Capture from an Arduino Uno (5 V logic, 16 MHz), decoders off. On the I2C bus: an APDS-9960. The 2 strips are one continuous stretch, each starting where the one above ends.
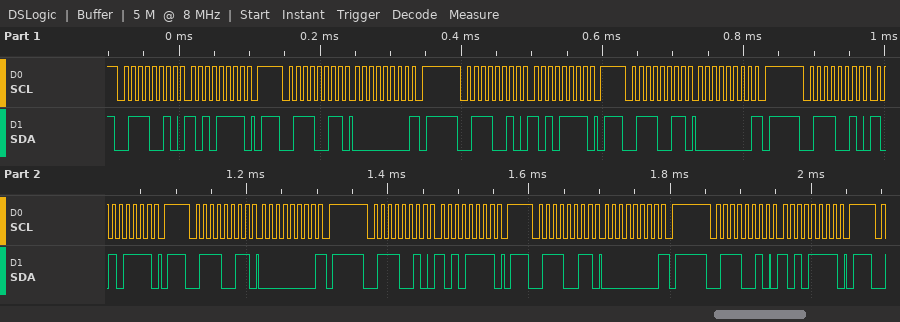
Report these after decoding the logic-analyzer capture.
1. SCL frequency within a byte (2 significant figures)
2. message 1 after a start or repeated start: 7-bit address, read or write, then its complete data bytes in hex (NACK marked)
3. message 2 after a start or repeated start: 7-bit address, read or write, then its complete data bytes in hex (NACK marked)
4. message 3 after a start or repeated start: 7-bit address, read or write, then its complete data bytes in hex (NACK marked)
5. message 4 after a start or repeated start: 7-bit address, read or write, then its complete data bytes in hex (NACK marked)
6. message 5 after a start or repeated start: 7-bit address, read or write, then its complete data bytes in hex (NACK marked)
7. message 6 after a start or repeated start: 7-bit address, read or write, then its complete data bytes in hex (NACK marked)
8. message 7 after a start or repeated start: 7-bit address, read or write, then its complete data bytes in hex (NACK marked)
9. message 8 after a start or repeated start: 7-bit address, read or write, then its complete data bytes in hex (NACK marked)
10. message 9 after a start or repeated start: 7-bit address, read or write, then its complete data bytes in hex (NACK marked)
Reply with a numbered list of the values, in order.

1. 100 kHz
2. 0x39 write: AF
3. 0x39 read: 00 NACK
4. 0x39 write: AF
5. 0x39 read: 00 NACK
6. 0x39 write: AF
7. 0x39 read: 00 NACK
8. 0x39 write: AF
9. 0x39 read: 00 NACK
10. 0x39 write: AF
